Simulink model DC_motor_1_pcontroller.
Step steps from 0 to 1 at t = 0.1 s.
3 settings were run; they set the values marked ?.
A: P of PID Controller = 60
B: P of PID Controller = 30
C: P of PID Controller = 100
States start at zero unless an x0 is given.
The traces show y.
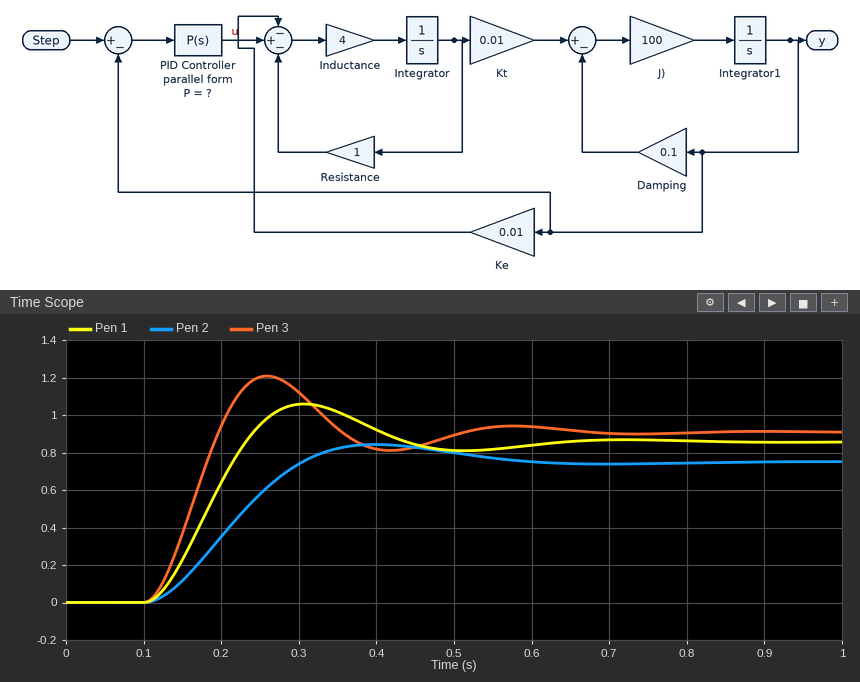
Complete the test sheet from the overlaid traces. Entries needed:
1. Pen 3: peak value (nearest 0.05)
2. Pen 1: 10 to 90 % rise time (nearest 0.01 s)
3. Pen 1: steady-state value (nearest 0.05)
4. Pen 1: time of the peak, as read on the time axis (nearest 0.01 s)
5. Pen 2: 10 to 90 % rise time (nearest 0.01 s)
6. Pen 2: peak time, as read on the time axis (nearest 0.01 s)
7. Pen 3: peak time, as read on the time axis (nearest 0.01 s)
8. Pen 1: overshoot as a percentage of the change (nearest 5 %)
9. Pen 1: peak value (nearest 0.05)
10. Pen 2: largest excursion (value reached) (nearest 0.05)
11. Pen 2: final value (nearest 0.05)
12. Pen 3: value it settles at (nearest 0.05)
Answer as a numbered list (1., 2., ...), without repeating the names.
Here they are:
1. 1.20
2. 0.09 s
3. 0.85
4. 0.31 s
5. 0.14 s
6. 0.40 s
7. 0.26 s
8. 25 %
9. 1.05
10. 0.85
11. 0.75
12. 0.90
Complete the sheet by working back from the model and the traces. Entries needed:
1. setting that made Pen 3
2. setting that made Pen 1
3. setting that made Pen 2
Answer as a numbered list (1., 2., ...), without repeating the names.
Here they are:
1. C
2. A
3. B
